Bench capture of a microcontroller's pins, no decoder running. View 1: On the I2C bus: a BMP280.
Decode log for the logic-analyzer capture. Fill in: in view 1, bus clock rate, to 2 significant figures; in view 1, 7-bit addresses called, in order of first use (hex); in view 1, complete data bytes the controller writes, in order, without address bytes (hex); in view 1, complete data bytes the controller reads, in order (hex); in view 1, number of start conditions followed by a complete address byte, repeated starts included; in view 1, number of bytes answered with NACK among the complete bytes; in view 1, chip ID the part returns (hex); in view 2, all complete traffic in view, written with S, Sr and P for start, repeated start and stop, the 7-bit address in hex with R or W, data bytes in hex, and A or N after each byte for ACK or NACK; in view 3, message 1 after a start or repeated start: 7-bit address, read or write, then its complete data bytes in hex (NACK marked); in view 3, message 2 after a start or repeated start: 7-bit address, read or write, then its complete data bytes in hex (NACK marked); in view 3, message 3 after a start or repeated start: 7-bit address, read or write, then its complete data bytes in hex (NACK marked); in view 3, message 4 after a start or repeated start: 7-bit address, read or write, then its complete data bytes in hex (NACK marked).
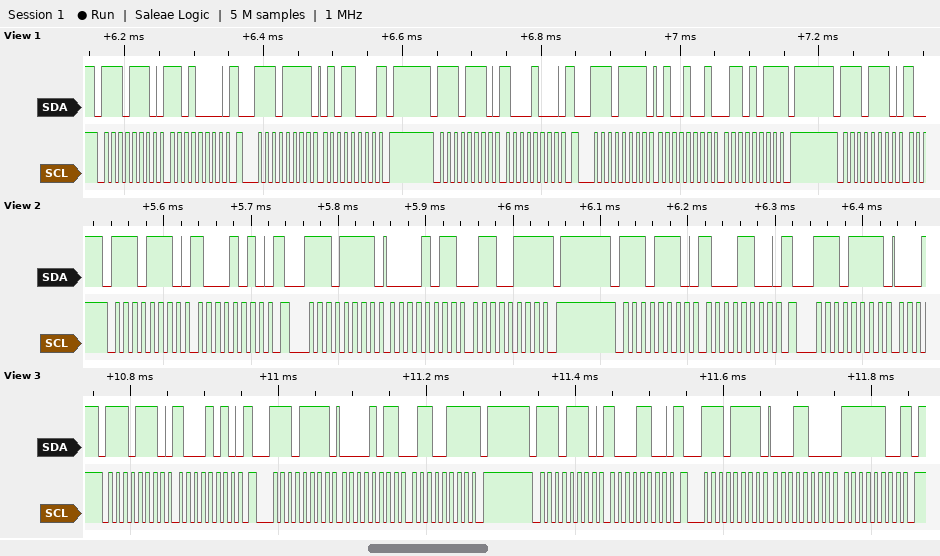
100 kHz
0x77
D0 88
58 49 6B
5
2
0x58
S 77W A 8A A Sr 77R A 0B A 67 N P S 77W A 8C A Sr 77R A
0x77 write: 8A
0x77 read: 0B 67 NACK
0x77 write: 8C
0x77 read: 18 FC NACK
